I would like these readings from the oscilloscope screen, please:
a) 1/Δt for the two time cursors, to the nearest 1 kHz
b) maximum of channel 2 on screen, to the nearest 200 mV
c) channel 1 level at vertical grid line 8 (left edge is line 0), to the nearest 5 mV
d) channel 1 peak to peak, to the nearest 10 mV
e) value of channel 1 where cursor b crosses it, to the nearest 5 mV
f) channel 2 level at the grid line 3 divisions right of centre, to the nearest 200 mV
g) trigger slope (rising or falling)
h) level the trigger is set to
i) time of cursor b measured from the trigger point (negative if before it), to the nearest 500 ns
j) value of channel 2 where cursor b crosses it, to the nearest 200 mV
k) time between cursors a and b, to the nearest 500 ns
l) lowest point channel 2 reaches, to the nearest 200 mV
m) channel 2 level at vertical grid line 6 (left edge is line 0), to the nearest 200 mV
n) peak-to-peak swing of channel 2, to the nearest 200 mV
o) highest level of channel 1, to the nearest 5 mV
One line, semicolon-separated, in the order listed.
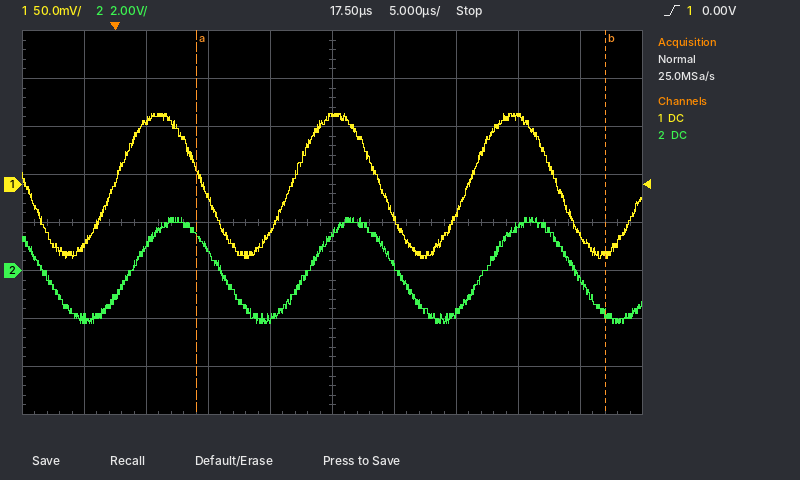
30 kHz; 2.2 V; 70 mV; 150 mV; -75 mV; 1.8 V; rising; 0.00 V; +39.5 µs; -1.8 V; 33.0 µs; -2.2 V; 200 mV; 4.4 V; 75 mV
